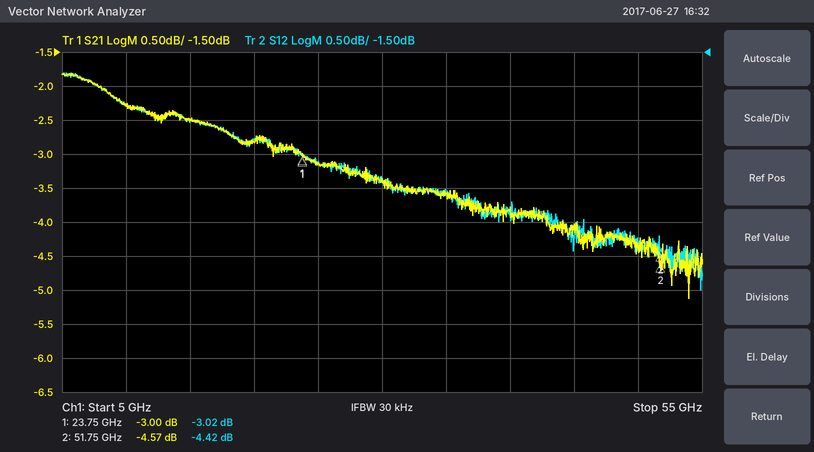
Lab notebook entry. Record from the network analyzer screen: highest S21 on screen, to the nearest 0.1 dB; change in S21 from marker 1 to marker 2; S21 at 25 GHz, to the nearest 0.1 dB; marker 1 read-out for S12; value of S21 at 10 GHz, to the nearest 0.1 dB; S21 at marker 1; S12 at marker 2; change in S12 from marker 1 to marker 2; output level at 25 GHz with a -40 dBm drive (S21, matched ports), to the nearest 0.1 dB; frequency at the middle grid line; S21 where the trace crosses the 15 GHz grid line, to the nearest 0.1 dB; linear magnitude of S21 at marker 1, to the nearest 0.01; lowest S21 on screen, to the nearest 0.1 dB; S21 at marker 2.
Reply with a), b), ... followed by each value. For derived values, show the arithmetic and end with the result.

a) -1.8 dB
b) -4.57 − (-3) = -1.57 dB
c) -3.1 dB
d) -3.02 dB
e) -2.3 dB
f) -3.00 dB
g) -4.42 dB
h) -4.42 − (-3.02) = -1.40 dB
i) -40 dBm + (-3.1 dB) = -43.1 dBm
j) 30 GHz
k) -2.5 dB
l) 10^(-3/20) ≈ 0.71
m) -5.1 dB
n) -4.57 dB
